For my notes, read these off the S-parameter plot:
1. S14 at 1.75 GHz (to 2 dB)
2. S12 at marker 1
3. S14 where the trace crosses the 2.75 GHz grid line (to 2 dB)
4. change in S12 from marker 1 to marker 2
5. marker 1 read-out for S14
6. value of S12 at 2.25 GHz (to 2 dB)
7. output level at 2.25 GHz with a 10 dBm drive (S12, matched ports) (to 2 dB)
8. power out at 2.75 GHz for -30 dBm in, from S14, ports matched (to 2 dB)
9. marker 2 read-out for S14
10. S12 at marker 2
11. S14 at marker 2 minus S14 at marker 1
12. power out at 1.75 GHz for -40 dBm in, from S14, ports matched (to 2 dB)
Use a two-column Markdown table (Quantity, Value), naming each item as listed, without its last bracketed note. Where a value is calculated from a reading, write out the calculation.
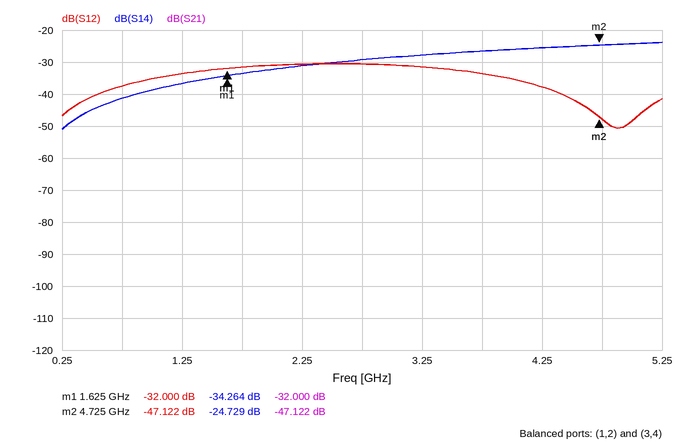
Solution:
| Quantity | Value |
|---|---|
| S14 at 1.75 GHz | -34 dB |
| S12 at marker 1 | -32.000 dB |
| S14 where the trace crosses the 2.75 GHz grid line | -30 dB |
| change in S12 from marker 1 to marker 2 | -47.122 − (-32) = -15.122 dB |
| marker 1 read-out for S14 | -34.264 dB |
| value of S12 at 2.25 GHz | -30 dB |
| output level at 2.25 GHz with a 10 dBm drive (S12, matched ports) | 10 dBm + (-30 dB) = -20 dBm |
| power out at 2.75 GHz for -30 dBm in, from S14, ports matched | -30 dBm + (-30 dB) = -60 dBm |
| marker 2 read-out for S14 | -24.729 dB |
| S12 at marker 2 | -47.122 dB |
| S14 at marker 2 minus S14 at marker 1 | -24.729 − (-34.264) = 9.535 dB |
| power out at 1.75 GHz for -40 dBm in, from S14, ports matched | -40 dBm + (-34 dB) = -74 dBm |
